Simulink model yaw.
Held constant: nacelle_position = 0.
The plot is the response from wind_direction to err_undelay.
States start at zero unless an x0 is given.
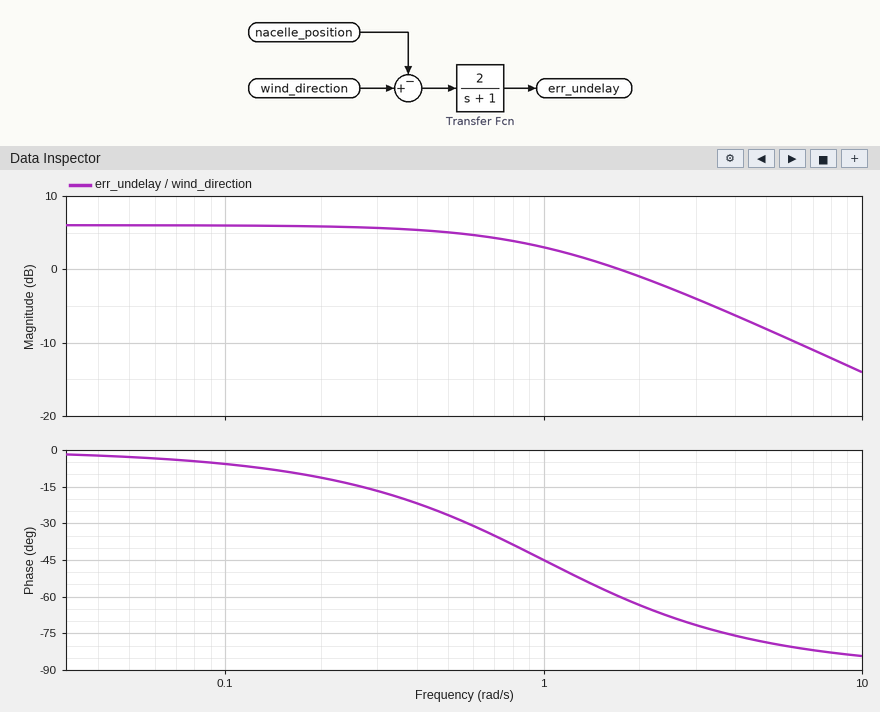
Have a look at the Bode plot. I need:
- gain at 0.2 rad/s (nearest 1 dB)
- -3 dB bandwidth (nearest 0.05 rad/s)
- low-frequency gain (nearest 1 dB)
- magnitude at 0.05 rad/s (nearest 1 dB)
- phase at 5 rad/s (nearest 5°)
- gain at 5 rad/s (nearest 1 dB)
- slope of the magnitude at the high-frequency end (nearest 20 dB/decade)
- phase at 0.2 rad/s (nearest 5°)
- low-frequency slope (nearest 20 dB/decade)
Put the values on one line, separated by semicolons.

6 dB; 1.00 rad/s; 6 dB; 6 dB; -80°; -8 dB; -20 dB/decade; -10°; 0 dB/decade
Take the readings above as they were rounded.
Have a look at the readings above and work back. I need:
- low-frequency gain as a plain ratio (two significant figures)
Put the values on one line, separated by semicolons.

2.0
